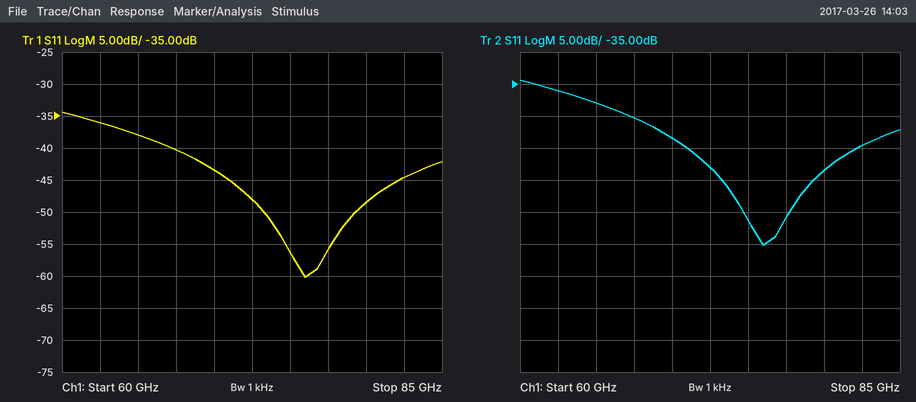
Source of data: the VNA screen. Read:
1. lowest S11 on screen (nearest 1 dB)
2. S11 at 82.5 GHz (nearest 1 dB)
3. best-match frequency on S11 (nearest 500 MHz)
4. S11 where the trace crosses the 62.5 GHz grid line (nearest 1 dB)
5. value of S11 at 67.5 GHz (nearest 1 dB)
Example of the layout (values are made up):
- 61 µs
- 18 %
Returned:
- -60 dB
- -45 dB
- 76.0 GHz
- -36 dB
- -40 dB
